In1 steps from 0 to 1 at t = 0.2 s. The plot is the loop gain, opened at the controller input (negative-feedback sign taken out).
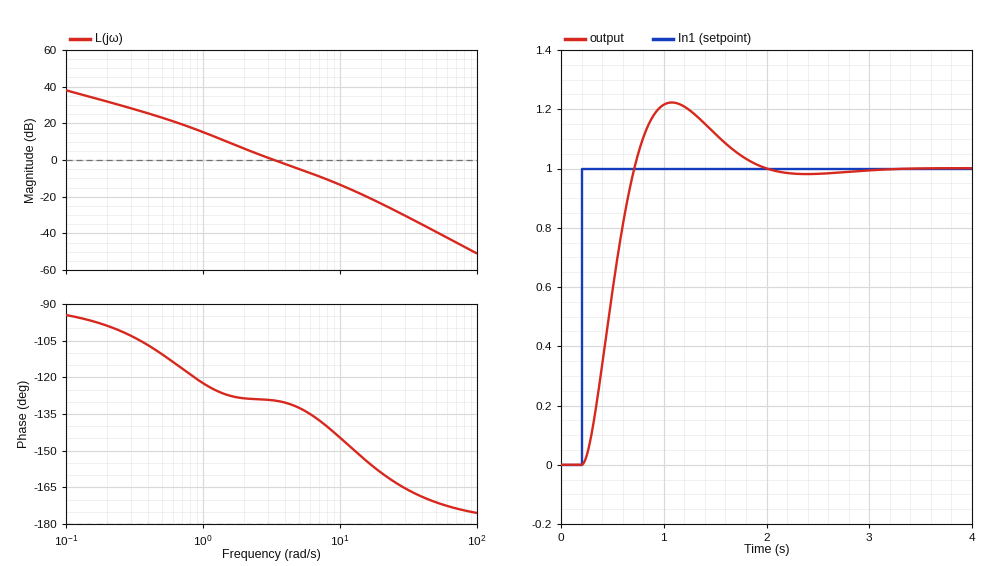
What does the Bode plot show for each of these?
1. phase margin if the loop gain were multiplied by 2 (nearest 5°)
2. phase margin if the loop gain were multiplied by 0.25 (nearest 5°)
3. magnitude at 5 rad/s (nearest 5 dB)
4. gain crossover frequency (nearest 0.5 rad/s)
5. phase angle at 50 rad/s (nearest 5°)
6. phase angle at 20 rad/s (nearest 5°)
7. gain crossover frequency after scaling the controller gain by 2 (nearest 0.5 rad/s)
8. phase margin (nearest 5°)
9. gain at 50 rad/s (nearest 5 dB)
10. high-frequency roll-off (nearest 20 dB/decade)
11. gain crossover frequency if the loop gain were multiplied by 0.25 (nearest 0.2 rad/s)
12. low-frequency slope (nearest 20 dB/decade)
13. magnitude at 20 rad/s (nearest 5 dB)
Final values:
45°
55°
-5 dB
3.5 rad/s
-170°
-160°
5.5 rad/s
50°
-40 dB
-40 dB/decade
1.2 rad/s
-20 dB/decade
-25 dB
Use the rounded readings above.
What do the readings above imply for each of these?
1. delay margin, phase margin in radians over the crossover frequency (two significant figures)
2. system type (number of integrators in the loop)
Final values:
0.25 s
1
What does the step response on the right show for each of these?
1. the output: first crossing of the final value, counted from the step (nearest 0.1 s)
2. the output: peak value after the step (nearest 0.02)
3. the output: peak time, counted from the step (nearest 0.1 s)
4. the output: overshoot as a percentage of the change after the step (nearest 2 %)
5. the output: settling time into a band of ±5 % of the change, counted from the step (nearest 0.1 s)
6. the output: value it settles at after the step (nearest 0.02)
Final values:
0.5 s
1.22
0.9 s
22 %
1.5 s
1.00
